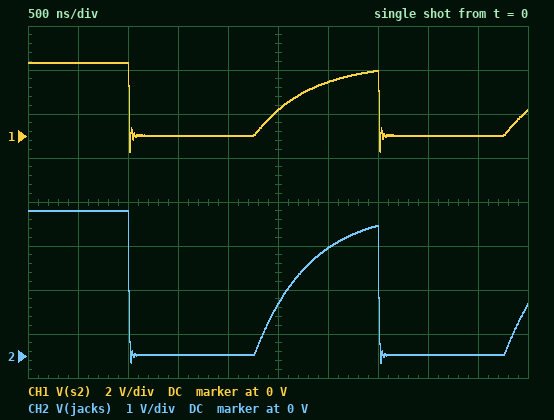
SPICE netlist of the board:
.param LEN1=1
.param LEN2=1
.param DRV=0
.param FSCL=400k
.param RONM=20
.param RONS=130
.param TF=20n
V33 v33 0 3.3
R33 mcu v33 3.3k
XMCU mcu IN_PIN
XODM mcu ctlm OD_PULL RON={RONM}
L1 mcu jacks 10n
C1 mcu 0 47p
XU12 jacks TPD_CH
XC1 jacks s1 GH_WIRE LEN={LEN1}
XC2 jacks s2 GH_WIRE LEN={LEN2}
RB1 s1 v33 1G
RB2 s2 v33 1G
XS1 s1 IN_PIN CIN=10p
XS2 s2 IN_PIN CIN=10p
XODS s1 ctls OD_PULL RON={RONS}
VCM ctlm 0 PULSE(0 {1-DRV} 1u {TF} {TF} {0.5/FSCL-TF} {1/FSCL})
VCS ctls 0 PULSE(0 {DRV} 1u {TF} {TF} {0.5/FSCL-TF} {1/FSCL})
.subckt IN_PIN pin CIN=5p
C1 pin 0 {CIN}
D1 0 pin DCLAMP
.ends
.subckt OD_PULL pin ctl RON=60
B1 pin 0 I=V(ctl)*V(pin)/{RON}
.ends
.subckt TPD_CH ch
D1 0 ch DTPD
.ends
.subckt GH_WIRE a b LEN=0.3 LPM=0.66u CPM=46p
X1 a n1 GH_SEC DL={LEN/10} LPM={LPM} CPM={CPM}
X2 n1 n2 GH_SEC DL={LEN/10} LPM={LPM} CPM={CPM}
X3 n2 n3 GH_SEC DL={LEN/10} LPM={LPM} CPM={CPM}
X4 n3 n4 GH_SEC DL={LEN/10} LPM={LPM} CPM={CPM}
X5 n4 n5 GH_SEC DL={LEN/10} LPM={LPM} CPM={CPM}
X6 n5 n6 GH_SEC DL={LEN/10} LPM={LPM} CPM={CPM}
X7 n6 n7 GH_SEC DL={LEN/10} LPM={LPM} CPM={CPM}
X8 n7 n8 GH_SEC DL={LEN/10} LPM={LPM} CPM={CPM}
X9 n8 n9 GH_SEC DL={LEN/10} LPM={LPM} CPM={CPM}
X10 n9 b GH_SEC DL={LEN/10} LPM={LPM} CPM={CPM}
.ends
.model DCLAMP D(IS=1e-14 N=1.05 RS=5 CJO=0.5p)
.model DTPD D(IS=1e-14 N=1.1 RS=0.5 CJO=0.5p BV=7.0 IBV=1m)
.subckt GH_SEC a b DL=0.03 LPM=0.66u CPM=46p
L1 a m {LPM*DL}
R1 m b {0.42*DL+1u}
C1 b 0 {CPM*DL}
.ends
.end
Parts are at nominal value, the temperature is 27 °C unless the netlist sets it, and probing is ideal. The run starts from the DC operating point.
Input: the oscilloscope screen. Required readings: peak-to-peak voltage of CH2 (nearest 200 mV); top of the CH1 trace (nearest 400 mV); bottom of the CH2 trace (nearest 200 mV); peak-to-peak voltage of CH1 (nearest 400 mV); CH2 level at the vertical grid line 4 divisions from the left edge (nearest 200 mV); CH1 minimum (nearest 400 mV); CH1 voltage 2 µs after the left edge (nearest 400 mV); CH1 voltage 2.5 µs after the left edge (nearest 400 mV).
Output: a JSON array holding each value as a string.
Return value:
["3.4 V", "3.2 V", "-200 mV", "4.0 V", "0 V", "-800 mV", "0 V", "1.2 V"]
